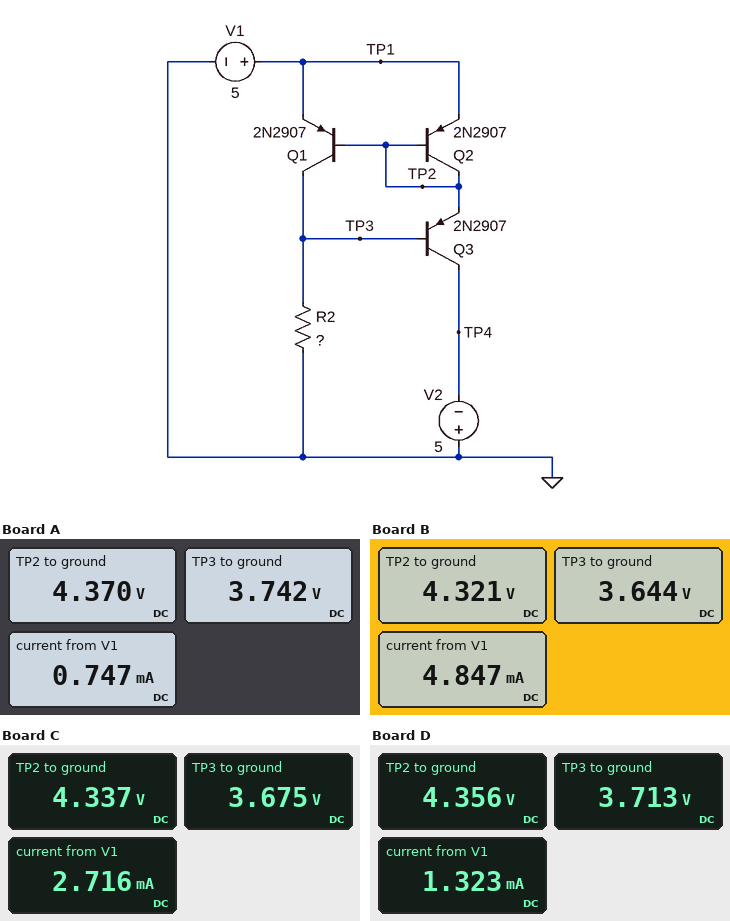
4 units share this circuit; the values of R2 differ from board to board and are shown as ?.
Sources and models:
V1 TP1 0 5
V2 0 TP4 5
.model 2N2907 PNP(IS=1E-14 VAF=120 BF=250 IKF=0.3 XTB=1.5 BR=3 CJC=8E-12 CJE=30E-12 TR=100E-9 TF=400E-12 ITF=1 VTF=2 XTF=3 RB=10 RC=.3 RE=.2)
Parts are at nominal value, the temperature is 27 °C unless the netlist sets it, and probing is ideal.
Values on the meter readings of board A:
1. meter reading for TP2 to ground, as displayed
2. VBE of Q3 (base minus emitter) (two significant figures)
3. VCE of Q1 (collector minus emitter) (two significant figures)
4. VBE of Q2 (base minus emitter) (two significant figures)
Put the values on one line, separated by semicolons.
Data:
4.370 V; -630 mV; -1.3 V; -630 mV
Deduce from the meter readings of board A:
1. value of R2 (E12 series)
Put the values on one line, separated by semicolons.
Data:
10 kΩ
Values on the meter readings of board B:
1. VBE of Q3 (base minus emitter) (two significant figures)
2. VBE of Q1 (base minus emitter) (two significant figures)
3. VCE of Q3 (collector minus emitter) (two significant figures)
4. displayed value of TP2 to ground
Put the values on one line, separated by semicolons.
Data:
-680 mV; -680 mV; -9.3 V; 4.321 V
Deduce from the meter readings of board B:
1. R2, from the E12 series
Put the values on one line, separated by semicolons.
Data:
1.5 kΩ
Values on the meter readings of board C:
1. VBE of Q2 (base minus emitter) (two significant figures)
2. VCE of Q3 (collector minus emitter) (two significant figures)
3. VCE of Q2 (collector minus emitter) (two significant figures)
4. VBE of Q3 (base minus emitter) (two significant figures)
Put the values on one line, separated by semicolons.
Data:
-660 mV; -9.3 V; -660 mV; -660 mV
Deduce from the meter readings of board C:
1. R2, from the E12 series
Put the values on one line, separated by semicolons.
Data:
2.7 kΩ
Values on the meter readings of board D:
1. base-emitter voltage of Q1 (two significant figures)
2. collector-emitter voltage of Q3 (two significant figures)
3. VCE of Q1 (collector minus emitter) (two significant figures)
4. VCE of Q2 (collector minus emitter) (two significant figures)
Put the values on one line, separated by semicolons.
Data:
-640 mV; -9.4 V; -1.3 V; -640 mV
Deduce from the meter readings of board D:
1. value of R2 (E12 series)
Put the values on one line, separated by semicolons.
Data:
5.6 kΩ
